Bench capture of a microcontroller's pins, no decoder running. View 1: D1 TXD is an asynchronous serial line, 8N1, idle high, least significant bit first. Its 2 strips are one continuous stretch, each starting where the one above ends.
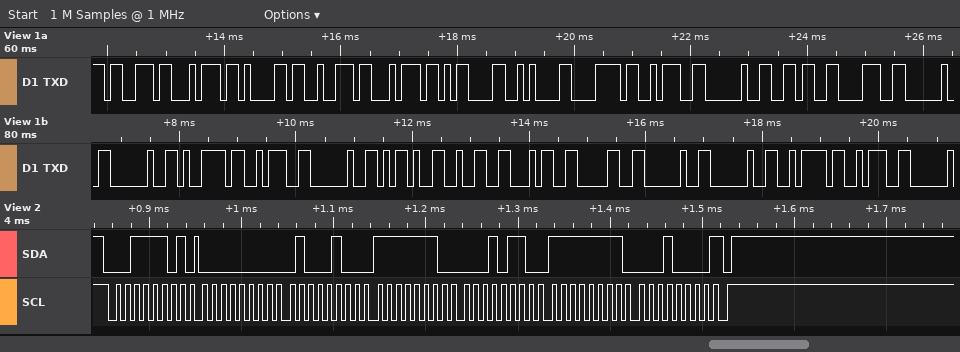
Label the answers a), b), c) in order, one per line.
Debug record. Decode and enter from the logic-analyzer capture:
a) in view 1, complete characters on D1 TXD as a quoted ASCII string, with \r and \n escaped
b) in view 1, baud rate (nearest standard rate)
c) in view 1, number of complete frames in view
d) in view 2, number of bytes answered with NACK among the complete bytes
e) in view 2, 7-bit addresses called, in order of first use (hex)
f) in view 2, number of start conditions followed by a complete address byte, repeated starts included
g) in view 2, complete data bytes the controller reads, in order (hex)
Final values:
a) "start\r\nx: 68  y: -240  z:"
b) 9600 baud
c) 25
d) 1
e) 0x1E
f) 1
g) 00 44 FE 16 FF 10
